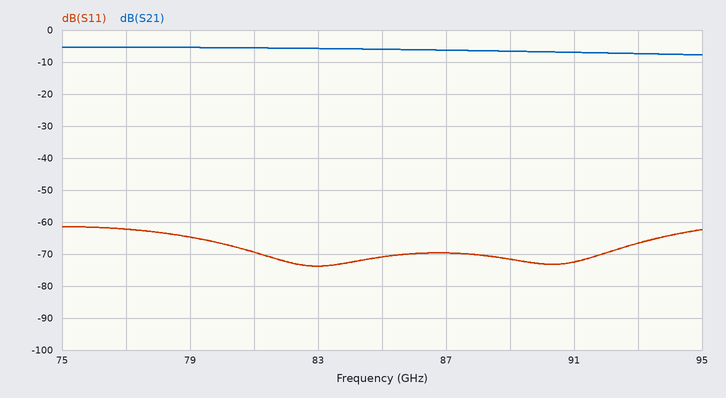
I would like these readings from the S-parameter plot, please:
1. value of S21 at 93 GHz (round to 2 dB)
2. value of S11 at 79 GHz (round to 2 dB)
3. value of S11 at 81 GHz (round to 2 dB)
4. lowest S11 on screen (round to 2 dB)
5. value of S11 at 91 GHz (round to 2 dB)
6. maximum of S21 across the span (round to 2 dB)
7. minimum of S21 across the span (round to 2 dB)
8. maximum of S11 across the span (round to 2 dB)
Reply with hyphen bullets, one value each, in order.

- -8 dB
- -64 dB
- -70 dB
- -74 dB
- -72 dB
- -6 dB
- -8 dB
- -62 dB
